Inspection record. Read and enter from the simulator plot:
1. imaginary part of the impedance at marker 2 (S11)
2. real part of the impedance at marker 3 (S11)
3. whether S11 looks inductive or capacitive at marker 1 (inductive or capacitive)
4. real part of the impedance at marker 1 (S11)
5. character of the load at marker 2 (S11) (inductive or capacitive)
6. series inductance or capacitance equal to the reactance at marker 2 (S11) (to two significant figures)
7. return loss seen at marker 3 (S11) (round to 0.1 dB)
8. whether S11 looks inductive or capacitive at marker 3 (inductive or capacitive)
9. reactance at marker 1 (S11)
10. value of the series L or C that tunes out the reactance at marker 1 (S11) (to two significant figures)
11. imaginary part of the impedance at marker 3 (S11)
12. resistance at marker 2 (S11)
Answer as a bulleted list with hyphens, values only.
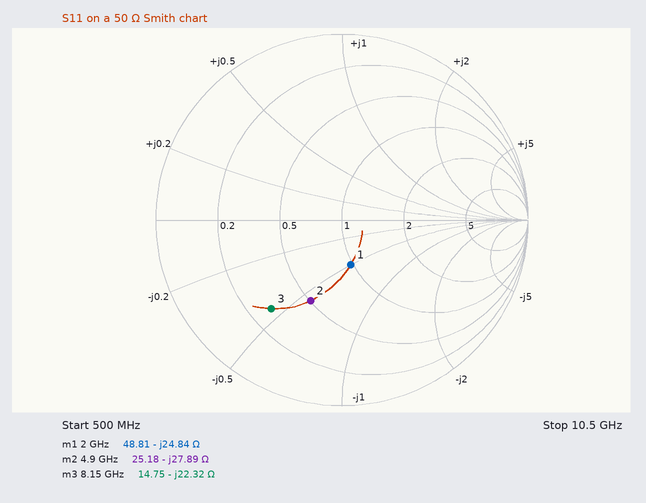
- -27.89 Ω
- 14.75 Ω
- capacitive
- 48.81 Ω
- capacitive
- 1.2 pF
- 4.3 dB
- capacitive
- -24.84 Ω
- 2.0 nH
- -22.32 Ω
- 25.18 Ω
